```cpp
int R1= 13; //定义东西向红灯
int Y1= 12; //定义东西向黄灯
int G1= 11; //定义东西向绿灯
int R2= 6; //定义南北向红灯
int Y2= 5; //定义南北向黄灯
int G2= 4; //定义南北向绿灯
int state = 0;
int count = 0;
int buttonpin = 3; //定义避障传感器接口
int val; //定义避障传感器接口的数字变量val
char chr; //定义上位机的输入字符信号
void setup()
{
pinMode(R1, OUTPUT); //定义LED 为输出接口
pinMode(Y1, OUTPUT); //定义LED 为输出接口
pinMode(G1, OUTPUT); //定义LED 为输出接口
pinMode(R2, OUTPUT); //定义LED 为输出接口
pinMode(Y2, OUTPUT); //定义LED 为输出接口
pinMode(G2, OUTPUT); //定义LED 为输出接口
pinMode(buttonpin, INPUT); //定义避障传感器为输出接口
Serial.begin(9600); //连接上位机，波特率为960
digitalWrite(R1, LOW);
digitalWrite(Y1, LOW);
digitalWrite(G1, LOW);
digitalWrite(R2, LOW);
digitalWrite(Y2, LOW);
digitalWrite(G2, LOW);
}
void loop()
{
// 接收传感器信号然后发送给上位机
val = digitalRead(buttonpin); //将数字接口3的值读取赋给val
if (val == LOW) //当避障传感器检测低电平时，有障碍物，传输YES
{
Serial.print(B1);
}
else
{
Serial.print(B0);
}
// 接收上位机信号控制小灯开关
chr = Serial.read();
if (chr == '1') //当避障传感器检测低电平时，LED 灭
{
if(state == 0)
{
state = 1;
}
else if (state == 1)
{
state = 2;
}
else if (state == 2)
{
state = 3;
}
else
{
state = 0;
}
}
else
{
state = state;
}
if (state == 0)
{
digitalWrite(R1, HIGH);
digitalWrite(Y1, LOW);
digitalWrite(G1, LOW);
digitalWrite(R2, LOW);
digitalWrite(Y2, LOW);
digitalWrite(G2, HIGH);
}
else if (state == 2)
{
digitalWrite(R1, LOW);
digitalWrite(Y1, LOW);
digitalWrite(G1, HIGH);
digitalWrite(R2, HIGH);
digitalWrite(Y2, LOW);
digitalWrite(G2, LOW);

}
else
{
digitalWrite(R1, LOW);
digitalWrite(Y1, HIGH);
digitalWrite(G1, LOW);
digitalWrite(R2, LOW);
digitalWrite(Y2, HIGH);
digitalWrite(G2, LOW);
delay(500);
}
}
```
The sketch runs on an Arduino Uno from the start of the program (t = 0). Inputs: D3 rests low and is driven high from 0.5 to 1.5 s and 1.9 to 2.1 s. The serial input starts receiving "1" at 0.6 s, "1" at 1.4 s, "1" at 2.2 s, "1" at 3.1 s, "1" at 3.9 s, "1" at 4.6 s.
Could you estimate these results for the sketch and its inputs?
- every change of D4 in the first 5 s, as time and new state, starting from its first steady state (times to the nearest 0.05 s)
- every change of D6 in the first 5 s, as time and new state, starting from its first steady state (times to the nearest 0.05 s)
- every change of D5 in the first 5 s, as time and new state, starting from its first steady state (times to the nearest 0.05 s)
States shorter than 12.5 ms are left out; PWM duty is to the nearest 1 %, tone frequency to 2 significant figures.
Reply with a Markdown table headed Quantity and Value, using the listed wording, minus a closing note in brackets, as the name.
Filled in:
| Quantity | Value |
|---|---|
| every change of D4 in the first 5 s, as time and new state, starting from its first steady state | 0 s high; 0.6 s low; 3.2 s high; 3.9 s low |
| every change of D6 in the first 5 s, as time and new state, starting from its first steady state | 0 s low; 1.6 s high; 2.2 s low; 4.9 s high |
| every change of D5 in the first 5 s, as time and new state, starting from its first steady state | 0 s low; 0.6 s high; 1.6 s low; 2.2 s high; 3.2 s low; 3.9 s high; 4.9 s low |
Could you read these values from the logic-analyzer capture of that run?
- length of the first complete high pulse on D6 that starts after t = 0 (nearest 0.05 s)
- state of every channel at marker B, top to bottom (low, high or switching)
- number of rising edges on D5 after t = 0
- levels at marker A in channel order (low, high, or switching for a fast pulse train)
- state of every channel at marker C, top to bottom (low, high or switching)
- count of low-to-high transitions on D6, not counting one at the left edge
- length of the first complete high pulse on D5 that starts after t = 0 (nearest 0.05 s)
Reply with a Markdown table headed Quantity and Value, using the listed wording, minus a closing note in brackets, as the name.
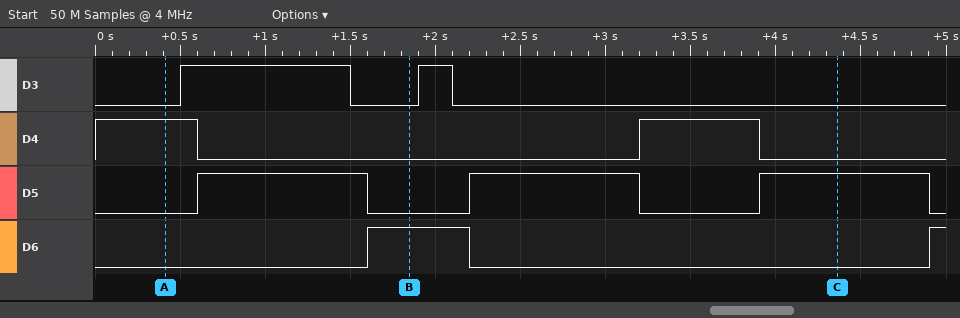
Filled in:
| Quantity | Value |
|---|---|
| length of the first complete high pulse on D6 that starts after t = 0 | 0.60 s |
| state of every channel at marker B, top to bottom | D3 low, D4 low, D5 low, D6 high |
| number of rising edges on D5 after t = 0 | 3 |
| levels at marker A in channel order | D3 low, D4 high, D5 low, D6 low |
| state of every channel at marker C, top to bottom | D3 low, D4 low, D5 high, D6 low |
| count of low-to-high transitions on D6, not counting one at the left edge | 2 |
| length of the first complete high pulse on D5 that starts after t = 0 | 1.00 s |
